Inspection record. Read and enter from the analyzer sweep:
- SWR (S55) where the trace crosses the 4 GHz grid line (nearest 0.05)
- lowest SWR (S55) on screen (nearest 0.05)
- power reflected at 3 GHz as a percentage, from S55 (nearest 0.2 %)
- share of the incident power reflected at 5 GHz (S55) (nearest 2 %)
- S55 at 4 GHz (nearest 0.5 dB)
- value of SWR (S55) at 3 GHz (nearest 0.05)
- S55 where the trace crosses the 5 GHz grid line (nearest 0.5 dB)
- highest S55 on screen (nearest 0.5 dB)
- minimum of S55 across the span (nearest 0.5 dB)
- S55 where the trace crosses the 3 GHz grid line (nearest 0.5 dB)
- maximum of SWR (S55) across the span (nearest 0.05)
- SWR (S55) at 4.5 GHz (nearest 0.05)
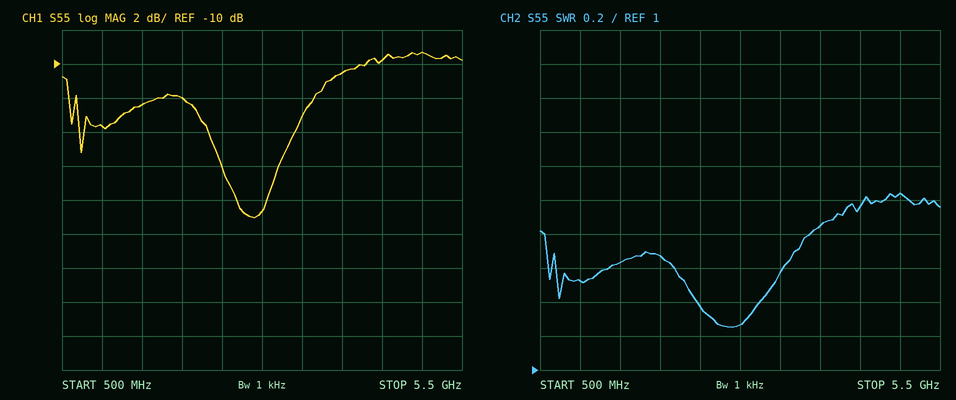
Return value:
1.85
1.25
1.4 %
12 %
-10.5 dB
1.25
-9.5 dB
-9.5 dB
-19.0 dB
-18.5 dB
2.05
1.95
